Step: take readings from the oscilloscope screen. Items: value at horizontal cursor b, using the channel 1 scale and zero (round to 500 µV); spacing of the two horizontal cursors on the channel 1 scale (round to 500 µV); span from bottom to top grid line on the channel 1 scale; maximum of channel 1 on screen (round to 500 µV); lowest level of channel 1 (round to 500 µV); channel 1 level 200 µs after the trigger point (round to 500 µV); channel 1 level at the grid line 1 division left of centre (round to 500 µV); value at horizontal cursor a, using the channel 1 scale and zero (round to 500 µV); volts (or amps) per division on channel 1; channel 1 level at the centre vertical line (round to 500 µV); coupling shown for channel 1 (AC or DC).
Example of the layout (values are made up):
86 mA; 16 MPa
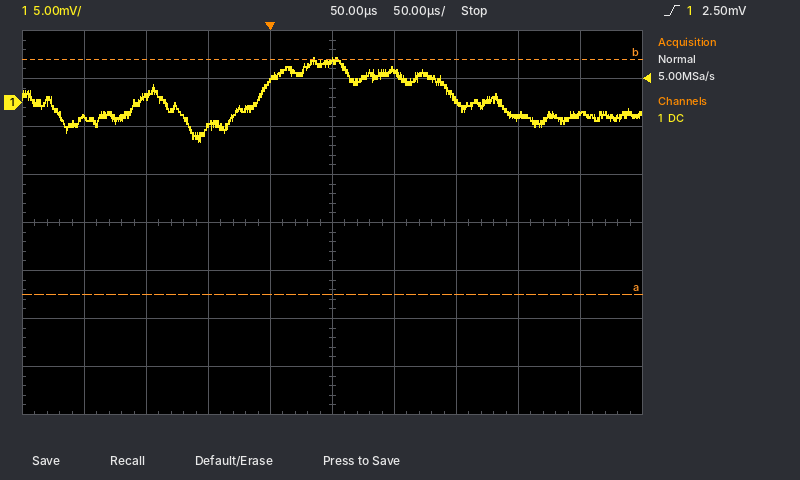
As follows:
4.5 mV; 24.5 mV; 40 mV; 4.5 mV; -4.0 mV; -1.5 mV; 2.5 mV; -20.0 mV; 5 mV; 4.5 mV; DC
